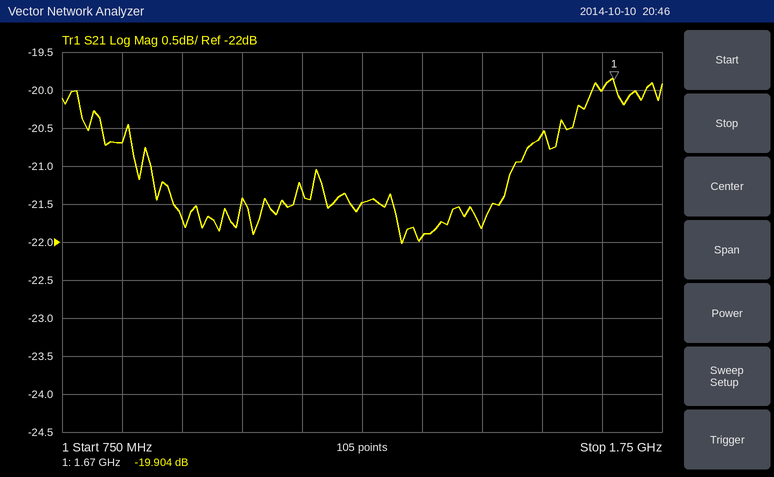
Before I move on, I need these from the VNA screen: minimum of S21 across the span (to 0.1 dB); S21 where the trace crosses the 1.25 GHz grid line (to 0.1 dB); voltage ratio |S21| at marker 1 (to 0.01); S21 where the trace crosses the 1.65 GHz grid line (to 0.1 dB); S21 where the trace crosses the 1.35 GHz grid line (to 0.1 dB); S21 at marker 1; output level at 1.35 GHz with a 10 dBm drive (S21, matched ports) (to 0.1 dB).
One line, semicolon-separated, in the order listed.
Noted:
-22.0 dB; -21.5 dB; 0.10; -20.0 dB; -21.9 dB; -19.904 dB; -11.9 dBm
